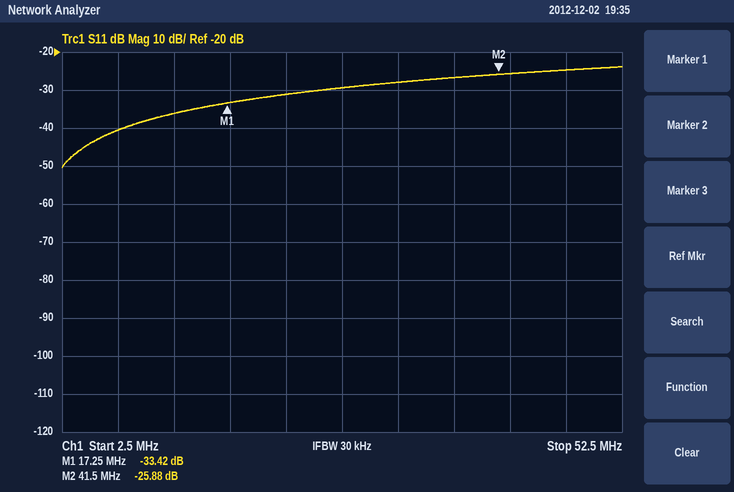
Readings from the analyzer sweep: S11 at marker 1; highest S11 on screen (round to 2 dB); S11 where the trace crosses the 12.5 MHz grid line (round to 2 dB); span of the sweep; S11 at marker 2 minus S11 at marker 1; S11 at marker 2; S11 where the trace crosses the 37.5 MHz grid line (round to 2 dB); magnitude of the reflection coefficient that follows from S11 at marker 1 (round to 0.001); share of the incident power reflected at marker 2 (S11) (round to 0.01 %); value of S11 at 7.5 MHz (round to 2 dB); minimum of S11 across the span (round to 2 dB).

-33.42 dB
-24 dB
-36 dB
50 MHz
7.54 dB
-25.88 dB
-26 dB
0.021
0.26 %
-40 dB
-50 dB
